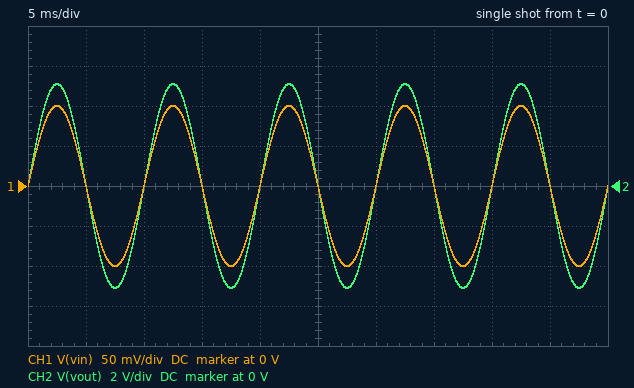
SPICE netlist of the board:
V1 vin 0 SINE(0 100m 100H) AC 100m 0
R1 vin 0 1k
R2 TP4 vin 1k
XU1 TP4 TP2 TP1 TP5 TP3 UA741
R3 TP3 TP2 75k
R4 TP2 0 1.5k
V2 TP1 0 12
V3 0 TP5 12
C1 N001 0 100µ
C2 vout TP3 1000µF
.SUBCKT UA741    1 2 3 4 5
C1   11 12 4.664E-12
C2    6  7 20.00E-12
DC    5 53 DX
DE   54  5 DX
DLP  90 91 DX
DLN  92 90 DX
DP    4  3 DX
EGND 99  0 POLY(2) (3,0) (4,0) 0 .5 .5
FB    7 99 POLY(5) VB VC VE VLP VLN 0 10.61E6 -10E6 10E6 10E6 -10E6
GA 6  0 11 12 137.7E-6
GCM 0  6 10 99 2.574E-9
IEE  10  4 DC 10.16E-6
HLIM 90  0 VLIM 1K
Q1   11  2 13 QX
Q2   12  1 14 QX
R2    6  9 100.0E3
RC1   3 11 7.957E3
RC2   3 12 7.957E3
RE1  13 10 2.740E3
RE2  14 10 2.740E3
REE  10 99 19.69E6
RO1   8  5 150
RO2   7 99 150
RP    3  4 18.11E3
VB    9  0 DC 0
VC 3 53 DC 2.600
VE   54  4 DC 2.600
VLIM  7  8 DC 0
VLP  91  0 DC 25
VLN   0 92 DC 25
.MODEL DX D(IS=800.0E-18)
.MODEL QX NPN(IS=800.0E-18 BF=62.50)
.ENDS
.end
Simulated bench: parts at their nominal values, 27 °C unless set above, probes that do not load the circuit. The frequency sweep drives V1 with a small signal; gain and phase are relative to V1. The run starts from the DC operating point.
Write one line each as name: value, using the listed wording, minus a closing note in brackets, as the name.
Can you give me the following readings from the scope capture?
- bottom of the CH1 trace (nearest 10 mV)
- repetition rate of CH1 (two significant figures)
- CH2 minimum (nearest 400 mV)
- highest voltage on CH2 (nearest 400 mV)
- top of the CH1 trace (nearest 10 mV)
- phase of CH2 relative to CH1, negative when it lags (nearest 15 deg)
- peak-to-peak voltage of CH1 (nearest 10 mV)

bottom of the CH1 trace: -100 mV
repetition rate of CH1: 100 Hz
CH2 minimum: -5.2 V
highest voltage on CH2: 5.2 V
top of the CH1 trace: 100 mV
phase of CH2 relative to CH1, negative when it lags: 0 deg
peak-to-peak voltage of CH1: 200 mV
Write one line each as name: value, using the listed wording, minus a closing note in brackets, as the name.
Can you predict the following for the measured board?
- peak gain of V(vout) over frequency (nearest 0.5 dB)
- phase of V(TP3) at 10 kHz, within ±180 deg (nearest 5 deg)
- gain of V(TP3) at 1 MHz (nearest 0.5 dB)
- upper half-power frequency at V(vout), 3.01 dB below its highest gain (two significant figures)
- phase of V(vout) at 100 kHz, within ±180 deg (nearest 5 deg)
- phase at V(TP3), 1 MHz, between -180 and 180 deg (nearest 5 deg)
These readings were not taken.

peak gain of V(vout) over frequency: 34.0 dB
phase of V(TP3) at 10 kHz, within ±180 deg: -25 deg
gain of V(TP3) at 1 MHz: 0 dB
upper half-power frequency at V(vout), 3.01 dB below its highest gain: 22 kHz
phase of V(vout) at 100 kHz, within ±180 deg: -80 deg
phase at V(TP3), 1 MHz, between -180 and 180 deg: -115 deg
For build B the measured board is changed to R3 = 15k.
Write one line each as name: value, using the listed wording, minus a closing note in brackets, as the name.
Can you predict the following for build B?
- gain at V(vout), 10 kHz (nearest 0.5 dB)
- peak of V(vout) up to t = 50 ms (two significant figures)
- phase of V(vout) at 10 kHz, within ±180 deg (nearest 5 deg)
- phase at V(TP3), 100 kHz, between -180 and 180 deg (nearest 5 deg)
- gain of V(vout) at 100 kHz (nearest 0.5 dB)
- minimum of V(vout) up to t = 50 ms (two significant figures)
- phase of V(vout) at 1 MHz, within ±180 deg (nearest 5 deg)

gain at V(vout), 10 kHz: 21.0 dB
peak of V(vout) up to t = 50 ms: 1.1 V
phase of V(vout) at 10 kHz, within ±180 deg: -5 deg
phase at V(TP3), 100 kHz, between -180 and 180 deg: -45 deg
gain of V(vout) at 100 kHz: 18.0 dB
minimum of V(vout) up to t = 50 ms: -1.1 V
phase of V(vout) at 1 MHz, within ±180 deg: -110 deg
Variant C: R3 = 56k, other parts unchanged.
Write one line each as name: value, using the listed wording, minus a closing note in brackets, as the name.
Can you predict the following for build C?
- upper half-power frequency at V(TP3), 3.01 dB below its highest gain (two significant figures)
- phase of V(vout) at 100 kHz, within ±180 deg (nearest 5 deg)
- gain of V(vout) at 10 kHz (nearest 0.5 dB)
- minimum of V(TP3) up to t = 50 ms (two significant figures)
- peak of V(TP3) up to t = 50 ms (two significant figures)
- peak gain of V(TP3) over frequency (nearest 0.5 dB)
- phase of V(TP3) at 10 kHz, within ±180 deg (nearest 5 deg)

upper half-power frequency at V(TP3), 3.01 dB below its highest gain: 29 kHz
phase of V(vout) at 100 kHz, within ±180 deg: -75 deg
gain of V(vout) at 10 kHz: 31.0 dB
minimum of V(TP3) up to t = 50 ms: -3.8 V
peak of V(TP3) up to t = 50 ms: 3.8 V
peak gain of V(TP3) over frequency: 31.5 dB
phase of V(TP3) at 10 kHz, within ±180 deg: -20 deg
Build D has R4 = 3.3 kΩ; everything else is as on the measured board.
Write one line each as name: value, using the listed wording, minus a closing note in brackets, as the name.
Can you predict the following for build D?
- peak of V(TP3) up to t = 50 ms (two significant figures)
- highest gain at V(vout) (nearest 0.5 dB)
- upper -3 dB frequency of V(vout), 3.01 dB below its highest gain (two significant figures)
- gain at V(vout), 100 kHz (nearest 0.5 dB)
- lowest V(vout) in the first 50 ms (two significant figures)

peak of V(TP3) up to t = 50 ms: 2.4 V
highest gain at V(vout): 27.5 dB
upper -3 dB frequency of V(vout), 3.01 dB below its highest gain: 47 kHz
gain at V(vout), 100 kHz: 20.0 dB
lowest V(vout) in the first 50 ms: -2.4 V
